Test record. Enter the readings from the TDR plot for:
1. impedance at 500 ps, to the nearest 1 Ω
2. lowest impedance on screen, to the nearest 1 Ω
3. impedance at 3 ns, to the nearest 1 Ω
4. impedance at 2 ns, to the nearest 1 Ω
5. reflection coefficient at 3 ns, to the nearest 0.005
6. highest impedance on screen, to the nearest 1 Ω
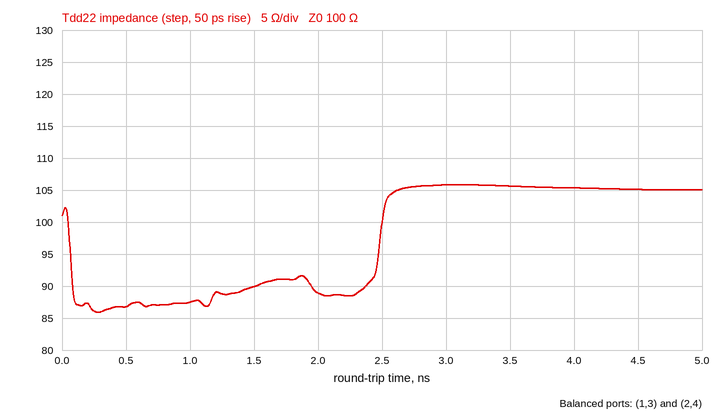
87 Ω
86 Ω
106 Ω
89 Ω
+0.030
106 Ω
